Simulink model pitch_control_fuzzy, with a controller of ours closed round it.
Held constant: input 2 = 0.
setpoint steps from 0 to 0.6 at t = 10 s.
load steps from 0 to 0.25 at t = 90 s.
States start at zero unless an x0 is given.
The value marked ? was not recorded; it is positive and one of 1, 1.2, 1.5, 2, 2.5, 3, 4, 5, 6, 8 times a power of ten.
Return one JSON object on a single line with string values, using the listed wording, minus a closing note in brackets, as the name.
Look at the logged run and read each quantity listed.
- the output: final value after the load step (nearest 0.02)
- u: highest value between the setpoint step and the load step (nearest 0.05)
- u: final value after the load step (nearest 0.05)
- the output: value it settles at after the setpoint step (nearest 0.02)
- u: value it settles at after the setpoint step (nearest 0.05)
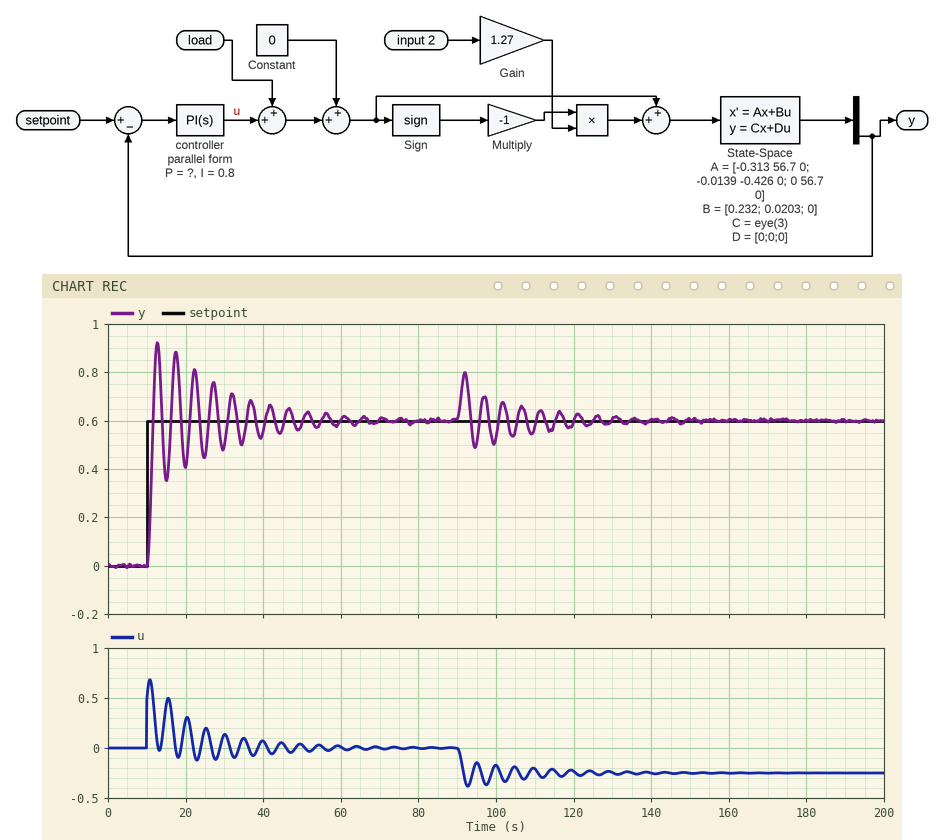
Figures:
{"the output: final value after the load step": "0.60", "u: highest value between the setpoint step and the load step": "0.70", "u: final value after the load step": "-0.25", "the output: value it settles at after the setpoint step": "0.60", "u: value it settles at after the setpoint step": "0.00"}
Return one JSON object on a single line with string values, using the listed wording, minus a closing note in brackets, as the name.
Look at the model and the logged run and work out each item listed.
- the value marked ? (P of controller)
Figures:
{"the value marked ?": "0.8"}
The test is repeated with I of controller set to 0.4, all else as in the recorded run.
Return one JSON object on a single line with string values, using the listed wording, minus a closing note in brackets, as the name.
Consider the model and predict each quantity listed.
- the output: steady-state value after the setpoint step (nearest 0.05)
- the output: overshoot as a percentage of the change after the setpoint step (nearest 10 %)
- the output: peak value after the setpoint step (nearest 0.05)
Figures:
{"the output: steady-state value after the setpoint step": "0.60", "the output: overshoot as a percentage of the change after the setpoint step": "20 %", "the output: peak value after the setpoint step": "0.75"}
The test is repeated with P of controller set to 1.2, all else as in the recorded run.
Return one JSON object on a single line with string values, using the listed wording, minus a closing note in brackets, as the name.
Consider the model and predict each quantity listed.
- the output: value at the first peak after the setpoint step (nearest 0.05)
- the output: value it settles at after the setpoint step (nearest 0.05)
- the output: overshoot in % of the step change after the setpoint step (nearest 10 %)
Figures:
{"the output: value at the first peak after the setpoint step": "0.90", "the output: value it settles at after the setpoint step": "0.60", "the output: overshoot in % of the step change after the setpoint step": "50 %"}
